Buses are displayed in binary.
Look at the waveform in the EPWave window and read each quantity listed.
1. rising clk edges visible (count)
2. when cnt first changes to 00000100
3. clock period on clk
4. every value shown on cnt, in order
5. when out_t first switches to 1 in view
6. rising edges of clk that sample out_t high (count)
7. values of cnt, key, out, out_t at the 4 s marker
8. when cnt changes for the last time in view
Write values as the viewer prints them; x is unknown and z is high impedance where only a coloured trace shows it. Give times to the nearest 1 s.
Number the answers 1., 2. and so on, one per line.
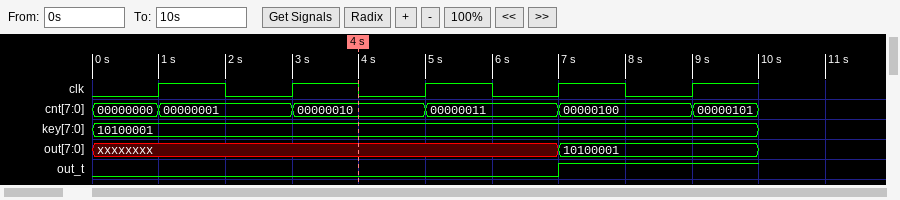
1. 5
2. 7 s
3. 2 s
4. 00000000, 00000001, 00000010, 00000011, 00000100, 00000101
5. 7 s
6. 1
7. cnt=00000010, key=10100001, out=xxxxxxxx, out_t=0
8. 9 s
